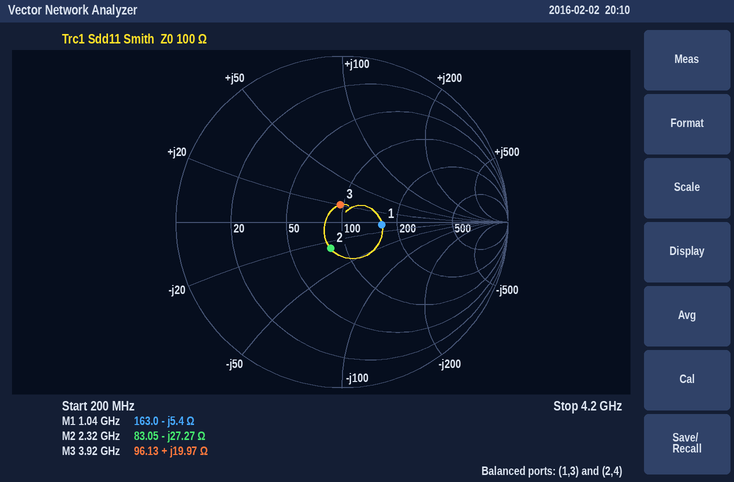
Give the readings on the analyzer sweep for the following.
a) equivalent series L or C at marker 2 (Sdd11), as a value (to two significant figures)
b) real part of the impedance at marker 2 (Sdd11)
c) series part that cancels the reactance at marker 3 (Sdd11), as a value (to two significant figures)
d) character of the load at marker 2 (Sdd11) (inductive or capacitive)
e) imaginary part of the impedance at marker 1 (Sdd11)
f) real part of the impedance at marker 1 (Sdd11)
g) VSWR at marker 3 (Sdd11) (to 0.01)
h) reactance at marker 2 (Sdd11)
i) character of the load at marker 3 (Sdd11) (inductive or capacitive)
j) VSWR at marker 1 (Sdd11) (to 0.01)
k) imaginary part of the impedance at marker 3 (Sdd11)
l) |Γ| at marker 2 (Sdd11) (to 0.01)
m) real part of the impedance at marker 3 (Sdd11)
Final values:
2.5 pF
83.05 Ω
2.0 pF
capacitive
-5.4 Ω
163.0 Ω
1.23
-27.27 Ω
inductive
1.63
+19.97 Ω
0.17
96.13 Ω
